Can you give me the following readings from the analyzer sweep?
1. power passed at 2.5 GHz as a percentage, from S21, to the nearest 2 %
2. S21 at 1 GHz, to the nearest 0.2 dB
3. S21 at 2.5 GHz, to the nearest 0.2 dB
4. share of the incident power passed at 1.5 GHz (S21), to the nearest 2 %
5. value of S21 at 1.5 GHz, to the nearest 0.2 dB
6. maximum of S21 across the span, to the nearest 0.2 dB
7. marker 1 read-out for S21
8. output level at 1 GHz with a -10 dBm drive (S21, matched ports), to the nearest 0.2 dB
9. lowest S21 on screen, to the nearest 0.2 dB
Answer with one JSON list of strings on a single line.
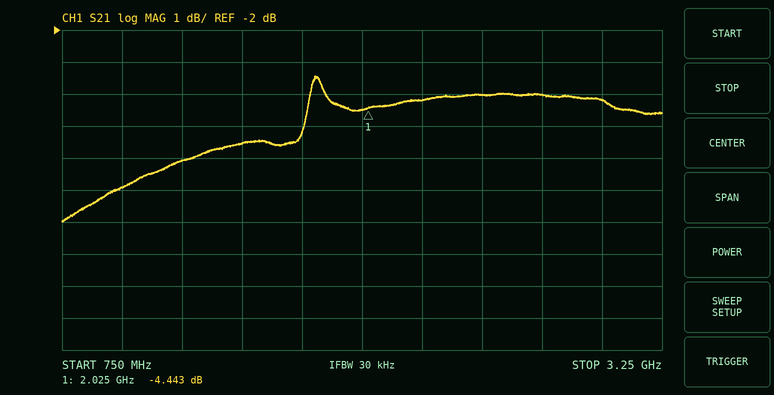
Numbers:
["40 %", "-7.0 dB", "-4.0 dB", "28 %", "-5.6 dB", "-3.4 dB", "-4.443 dB", "-17.0 dBm", "-8.0 dB"]
